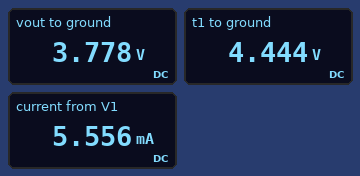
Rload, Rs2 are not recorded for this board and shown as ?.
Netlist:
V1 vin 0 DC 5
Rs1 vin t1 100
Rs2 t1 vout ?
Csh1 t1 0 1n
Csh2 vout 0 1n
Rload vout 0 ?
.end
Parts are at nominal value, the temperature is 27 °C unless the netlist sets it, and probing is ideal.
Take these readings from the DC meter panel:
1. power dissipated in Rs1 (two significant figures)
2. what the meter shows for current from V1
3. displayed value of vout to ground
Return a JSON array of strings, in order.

["3.1 mW", "5.556 mA", "3.778 V"]
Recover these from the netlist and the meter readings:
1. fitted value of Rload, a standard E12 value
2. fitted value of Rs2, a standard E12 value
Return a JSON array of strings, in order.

["680 Ω", "120 Ω"]
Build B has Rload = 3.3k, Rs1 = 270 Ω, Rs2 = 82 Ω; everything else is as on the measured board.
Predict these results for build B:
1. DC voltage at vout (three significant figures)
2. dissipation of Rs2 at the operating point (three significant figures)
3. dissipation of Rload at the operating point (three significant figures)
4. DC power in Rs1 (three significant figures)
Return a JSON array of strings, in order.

["4.52 V", "154 µW", "6.19 mW", "506 µW"]
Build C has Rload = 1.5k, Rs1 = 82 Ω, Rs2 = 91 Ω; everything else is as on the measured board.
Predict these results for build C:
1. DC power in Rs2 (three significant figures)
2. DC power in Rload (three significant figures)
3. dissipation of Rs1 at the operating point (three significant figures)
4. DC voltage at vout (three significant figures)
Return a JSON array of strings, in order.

["813 µW", "13.4 mW", "732 µW", "4.48 V"]
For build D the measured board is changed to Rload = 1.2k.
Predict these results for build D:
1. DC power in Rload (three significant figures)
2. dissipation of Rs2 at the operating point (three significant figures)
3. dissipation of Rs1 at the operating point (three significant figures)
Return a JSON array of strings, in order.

["14.9 mW", "1.49 mW", "1.24 mW"]
